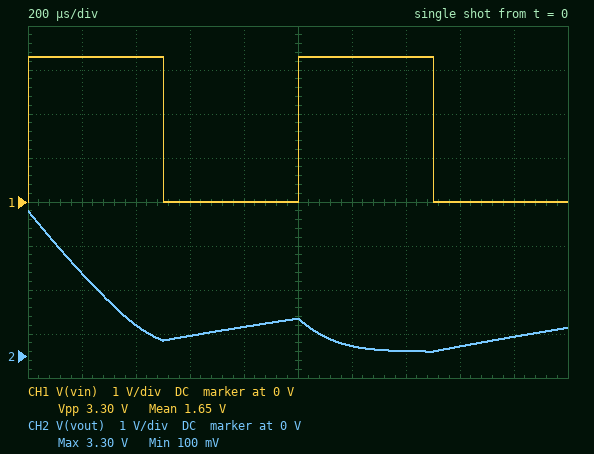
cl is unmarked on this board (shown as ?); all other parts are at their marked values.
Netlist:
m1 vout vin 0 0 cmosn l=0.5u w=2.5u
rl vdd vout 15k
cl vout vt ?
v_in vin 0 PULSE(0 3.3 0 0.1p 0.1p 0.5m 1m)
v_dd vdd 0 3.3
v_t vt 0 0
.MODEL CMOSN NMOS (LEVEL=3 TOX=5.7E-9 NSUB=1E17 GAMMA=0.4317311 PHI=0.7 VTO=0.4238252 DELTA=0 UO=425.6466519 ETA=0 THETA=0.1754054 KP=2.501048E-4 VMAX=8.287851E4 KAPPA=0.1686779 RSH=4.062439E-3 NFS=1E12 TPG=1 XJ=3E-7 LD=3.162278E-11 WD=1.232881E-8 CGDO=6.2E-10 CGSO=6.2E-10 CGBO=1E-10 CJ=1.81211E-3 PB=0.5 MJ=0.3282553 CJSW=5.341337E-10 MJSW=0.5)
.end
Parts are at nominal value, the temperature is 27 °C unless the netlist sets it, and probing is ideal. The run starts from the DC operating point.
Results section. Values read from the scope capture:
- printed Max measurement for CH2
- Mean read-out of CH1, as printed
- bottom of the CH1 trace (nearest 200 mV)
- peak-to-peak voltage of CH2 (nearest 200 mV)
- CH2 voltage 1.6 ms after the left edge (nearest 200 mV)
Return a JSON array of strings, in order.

["3.30 V", "1.65 V", "0 V", "3.2 V", "200 mV"]
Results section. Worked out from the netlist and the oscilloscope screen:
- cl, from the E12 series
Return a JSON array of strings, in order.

["180 nF"]
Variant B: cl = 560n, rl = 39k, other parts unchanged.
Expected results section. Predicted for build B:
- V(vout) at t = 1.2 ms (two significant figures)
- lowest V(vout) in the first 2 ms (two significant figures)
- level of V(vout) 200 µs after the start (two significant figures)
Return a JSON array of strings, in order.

["1.7 V", "1.1 V", "2.8 V"]
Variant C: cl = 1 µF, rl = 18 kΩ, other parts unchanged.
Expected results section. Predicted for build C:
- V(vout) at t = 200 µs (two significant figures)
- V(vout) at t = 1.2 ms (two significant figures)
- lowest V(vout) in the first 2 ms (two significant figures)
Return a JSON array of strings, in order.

["3.0 V", "2.4 V", "2.0 V"]
